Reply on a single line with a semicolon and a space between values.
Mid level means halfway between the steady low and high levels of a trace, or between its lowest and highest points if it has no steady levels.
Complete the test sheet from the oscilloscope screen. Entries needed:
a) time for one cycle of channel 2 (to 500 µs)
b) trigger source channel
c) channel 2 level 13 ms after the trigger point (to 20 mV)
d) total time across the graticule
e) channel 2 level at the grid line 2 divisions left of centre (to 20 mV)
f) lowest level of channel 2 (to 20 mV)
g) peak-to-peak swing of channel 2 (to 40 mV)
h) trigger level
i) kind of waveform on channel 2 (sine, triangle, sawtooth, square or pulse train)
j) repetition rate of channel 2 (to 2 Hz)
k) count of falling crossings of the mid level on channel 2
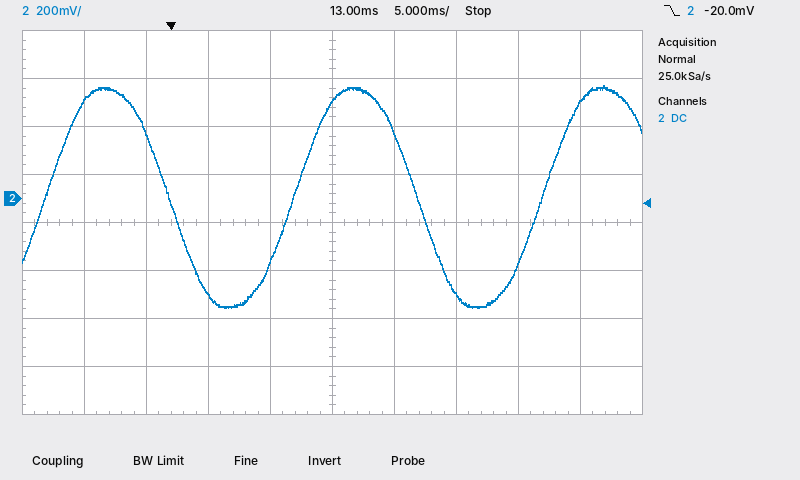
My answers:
20.0 ms; channel 2; 400 mV; 50 ms; -400 mV; -460 mV; 920 mV; -20.0 mV; sine; 50 Hz; 2
